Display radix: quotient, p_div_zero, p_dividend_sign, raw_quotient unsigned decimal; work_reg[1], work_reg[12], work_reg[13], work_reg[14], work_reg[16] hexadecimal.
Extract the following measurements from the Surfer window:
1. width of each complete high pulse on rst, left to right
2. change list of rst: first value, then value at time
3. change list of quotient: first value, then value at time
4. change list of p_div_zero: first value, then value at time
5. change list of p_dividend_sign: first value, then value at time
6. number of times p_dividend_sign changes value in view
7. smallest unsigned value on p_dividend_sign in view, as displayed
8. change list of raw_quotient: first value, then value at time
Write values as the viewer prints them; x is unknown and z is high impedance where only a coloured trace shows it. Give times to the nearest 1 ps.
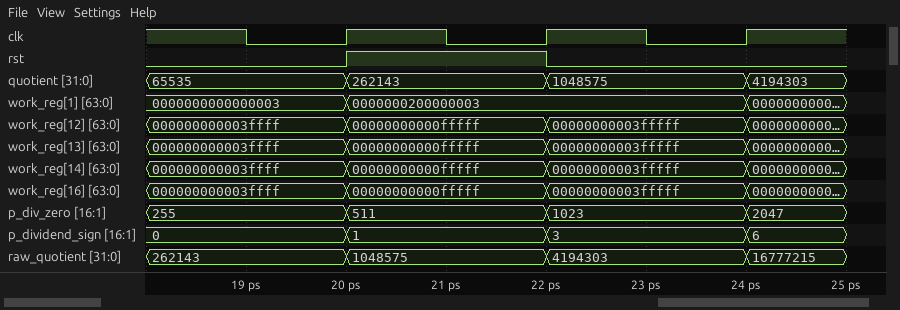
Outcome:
2 ps
0, 1 at 20 ps, 0 at 22 ps
65535, 262143 at 20 ps, 1048575 at 22 ps, 4194303 at 24 ps
255, 511 at 20 ps, 1023 at 22 ps, 2047 at 24 ps
0, 1 at 20 ps, 3 at 22 ps, 6 at 24 ps
3
0
262143, 1048575 at 20 ps, 4194303 at 22 ps, 16777215 at 24 ps
